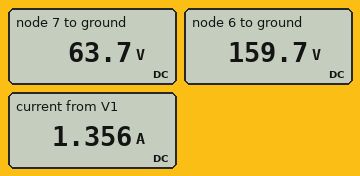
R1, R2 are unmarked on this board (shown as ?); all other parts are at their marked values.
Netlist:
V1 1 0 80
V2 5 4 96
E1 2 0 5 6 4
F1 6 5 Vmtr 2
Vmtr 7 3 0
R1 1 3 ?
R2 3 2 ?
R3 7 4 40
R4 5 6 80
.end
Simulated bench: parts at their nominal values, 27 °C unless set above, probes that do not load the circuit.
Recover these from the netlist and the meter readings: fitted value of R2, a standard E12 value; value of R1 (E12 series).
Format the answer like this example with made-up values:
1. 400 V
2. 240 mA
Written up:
1. 47 Ω
2. 12 Ω
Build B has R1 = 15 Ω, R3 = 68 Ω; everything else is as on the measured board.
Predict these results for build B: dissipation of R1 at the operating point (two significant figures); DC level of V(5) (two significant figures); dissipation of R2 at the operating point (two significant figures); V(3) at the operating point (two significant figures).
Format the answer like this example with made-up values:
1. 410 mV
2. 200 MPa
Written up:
1. 25 W
2. 160 V
3. 78 W
4. 61 V
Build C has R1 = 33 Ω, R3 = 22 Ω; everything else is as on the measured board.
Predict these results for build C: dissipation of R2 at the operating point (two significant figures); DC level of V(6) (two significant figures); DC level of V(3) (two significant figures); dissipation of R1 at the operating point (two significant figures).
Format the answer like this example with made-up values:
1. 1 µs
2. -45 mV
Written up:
1. 47 W
2. 140 V
3. 47 V
4. 33 W
